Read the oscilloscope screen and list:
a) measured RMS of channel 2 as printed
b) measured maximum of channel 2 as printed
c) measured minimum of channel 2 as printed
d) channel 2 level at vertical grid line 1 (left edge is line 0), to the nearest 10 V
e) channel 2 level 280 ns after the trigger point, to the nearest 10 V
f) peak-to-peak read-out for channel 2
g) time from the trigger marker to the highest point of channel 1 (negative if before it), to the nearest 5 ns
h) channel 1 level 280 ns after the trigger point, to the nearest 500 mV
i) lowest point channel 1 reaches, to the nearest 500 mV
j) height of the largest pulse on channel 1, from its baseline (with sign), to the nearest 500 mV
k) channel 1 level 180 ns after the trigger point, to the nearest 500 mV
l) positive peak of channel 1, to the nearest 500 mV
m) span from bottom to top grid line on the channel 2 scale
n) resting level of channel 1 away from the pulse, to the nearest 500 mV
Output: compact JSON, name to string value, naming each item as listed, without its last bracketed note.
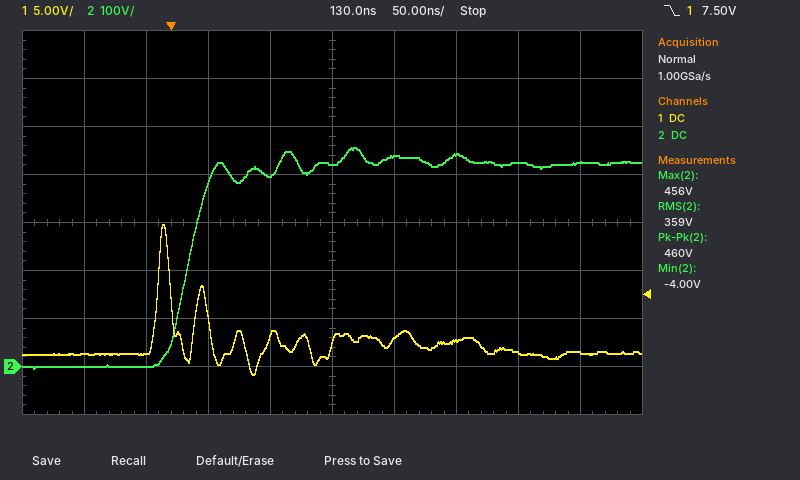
{"measured RMS of channel 2 as printed": "359 V", "measured maximum of channel 2 as printed": "456 V", "measured minimum of channel 2 as printed": "-4.00 V", "channel 2 level at vertical grid line 1 (left edge is line 0), to the nearest 10 V": "0 V", "channel 2 level 280 ns after the trigger point, to the nearest 10 V": "420 V", "peak-to-peak read-out for channel 2": "460 V", "time from the trigger marker to the highest point of channel 1 (negative if before it), to the nearest 5 ns": "-5 ns", "channel 1 level 280 ns after the trigger point, to the nearest 500 mV": "1.5 V", "lowest point channel 1 reaches, to the nearest 500 mV": "-1.0 V", "height of the largest pulse on channel 1, from its baseline (with sign), to the nearest 500 mV": "+13.5 V", "channel 1 level 180 ns after the trigger point, to the nearest 500 mV": "3.0 V", "positive peak of channel 1, to the nearest 500 mV": "15.0 V", "span from bottom to top grid line on the channel 2 scale": "800 V", "resting level of channel 1 away from the pulse, to the nearest 500 mV": "1.5 V"}
